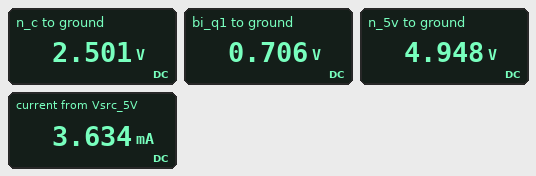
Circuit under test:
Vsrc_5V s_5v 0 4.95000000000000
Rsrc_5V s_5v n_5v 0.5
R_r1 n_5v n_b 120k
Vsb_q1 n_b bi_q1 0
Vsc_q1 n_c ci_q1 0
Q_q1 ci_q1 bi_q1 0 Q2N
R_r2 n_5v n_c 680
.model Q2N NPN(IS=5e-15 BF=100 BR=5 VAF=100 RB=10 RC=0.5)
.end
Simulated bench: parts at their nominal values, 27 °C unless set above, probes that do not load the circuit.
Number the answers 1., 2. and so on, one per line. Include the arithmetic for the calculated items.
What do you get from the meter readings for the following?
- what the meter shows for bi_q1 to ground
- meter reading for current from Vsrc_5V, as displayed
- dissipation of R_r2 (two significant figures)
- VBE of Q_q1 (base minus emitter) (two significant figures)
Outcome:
1. 0.706 V
2. 3.634 mA
3. (4.948 V - 2.501 V)^2 / 680 Ω = 8.8 mW
4. 706 mV = 710 mV
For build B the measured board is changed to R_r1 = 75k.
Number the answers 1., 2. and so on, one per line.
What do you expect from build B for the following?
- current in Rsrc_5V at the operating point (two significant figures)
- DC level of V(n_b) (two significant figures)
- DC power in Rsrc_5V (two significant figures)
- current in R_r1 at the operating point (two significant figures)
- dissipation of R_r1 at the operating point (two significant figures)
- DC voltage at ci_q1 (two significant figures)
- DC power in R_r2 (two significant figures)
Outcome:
1. 5.7 mA
2. 720 mV
3. 16 µW
4. 56 µA
5. 240 µW
6. 1.1 V
7. 22 mW
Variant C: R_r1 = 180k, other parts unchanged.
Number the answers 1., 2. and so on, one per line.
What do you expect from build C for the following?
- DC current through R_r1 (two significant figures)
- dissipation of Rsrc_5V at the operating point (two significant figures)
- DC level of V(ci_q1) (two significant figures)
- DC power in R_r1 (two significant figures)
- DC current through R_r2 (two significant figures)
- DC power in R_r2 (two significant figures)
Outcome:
1. 24 µA
2. 3.0 µW
3. 3.3 V
4. 100 µW
5. 2.4 mA
6. 4.0 mW
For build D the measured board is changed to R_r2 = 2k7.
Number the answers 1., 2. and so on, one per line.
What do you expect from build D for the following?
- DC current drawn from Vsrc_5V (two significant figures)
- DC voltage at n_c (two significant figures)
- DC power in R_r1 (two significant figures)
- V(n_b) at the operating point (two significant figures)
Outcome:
1. 1.8 mA
2. 82 mV
3. 150 µW
4. 690 mV
